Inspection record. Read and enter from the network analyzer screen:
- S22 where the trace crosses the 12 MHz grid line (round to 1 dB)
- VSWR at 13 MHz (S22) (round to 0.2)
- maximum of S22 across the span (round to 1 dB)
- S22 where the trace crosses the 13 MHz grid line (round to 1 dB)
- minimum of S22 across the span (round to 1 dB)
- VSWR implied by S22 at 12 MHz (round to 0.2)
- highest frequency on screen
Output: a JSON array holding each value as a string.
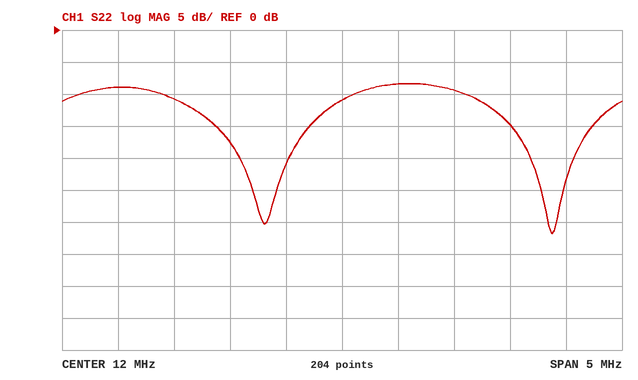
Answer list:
["-11 dB", "2.0", "-8 dB", "-9 dB", "-32 dB", "1.8", "14.5 MHz"]
